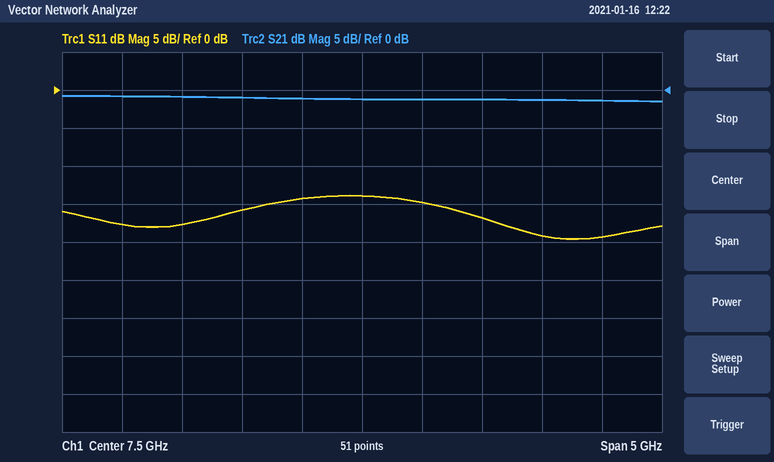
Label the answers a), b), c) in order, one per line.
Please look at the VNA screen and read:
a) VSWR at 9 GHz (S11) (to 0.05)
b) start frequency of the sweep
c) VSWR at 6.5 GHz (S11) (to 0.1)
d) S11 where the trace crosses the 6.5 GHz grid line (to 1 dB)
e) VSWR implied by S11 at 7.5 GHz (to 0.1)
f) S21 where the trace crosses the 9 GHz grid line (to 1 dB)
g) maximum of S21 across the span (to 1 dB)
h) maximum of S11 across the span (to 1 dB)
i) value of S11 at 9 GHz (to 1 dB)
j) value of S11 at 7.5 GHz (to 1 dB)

a) 1.25
b) 5 GHz
c) 1.4
d) -16 dB
e) 1.5
f) -1 dB
g) -1 dB
h) -14 dB
i) -19 dB
j) -14 dB
